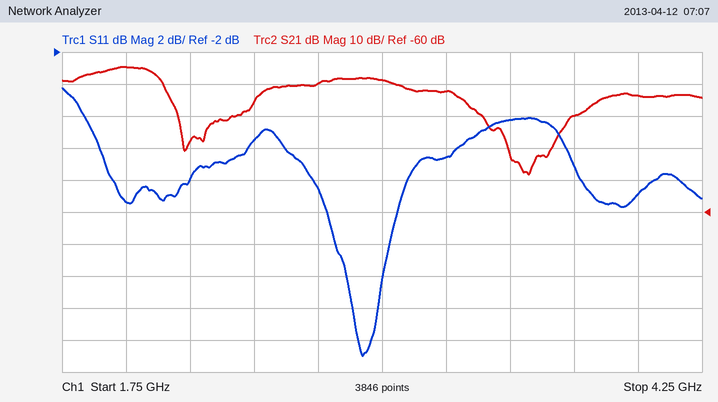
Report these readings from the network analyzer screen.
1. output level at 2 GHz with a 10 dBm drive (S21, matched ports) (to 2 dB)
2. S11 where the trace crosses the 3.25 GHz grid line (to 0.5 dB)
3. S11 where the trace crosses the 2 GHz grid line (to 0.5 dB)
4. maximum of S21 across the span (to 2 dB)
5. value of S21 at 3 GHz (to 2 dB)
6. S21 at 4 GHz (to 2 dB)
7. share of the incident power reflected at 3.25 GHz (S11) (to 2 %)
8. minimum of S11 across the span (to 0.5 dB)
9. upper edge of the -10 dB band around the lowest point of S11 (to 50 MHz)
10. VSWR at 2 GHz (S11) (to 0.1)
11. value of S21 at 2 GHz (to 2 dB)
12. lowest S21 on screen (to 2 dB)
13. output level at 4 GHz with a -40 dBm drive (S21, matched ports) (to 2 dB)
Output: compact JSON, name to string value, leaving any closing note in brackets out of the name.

{"output level at 2 GHz with a 10 dBm drive (S21, matched ports)": "-4 dBm", "S11 where the trace crosses the 3.25 GHz grid line": "-8.5 dB", "S11 where the trace crosses the 2 GHz grid line": "-11.5 dB", "maximum of S21 across the span": "-14 dB", "value of S21 at 3 GHz": "-18 dB", "S21 at 4 GHz": "-24 dB", "share of the incident power reflected at 3.25 GHz (S11)": "14 %", "minimum of S11 across the span": "-21.0 dB", "upper edge of the -10 dB band around the lowest point of S11": "3.10 GHz", "VSWR at 2 GHz (S11)": "1.7", "value of S21 at 2 GHz": "-14 dB", "lowest S21 on screen": "-48 dB", "output level at 4 GHz with a -40 dBm drive (S21, matched ports)": "-64 dBm"}
